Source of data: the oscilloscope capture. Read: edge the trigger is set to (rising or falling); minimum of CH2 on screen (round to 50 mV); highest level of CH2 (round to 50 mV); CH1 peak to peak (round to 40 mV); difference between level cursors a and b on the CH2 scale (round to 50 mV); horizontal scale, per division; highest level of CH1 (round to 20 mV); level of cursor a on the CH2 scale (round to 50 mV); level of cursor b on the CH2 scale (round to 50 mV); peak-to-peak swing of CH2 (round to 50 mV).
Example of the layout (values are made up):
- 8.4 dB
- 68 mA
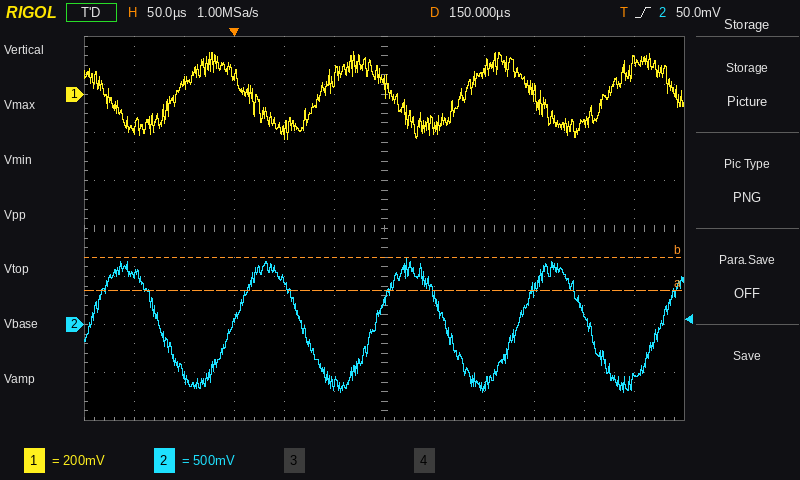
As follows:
- rising
- -700 mV
- 700 mV
- 360 mV
- 350 mV
- 50 µs
- 180 mV
- 350 mV
- 700 mV
- 1.40 V
